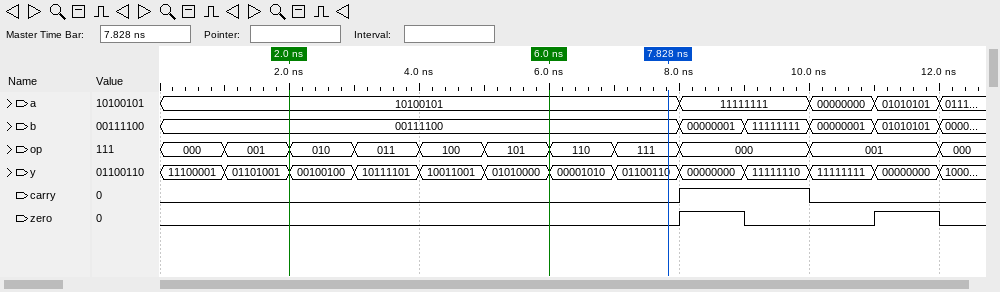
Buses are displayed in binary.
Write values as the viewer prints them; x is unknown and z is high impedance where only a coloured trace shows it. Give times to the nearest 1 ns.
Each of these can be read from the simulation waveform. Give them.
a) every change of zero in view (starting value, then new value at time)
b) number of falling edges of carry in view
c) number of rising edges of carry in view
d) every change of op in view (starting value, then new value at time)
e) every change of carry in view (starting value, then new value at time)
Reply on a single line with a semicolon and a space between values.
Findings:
0, 1 at 8 ns, 0 at 9 ns, 1 at 11 ns, 0 at 12 ns; 1; 1; 000, 001 at 1 ns, 010 at 2 ns, 011 at 3 ns, 100 at 4 ns, 101 at 5 ns, 110 at 6 ns, 111 at 7 ns, 000 at 8 ns, 001 at 10 ns, 000 at 12 ns; 0, 1 at 8 ns, 0 at 10 ns
